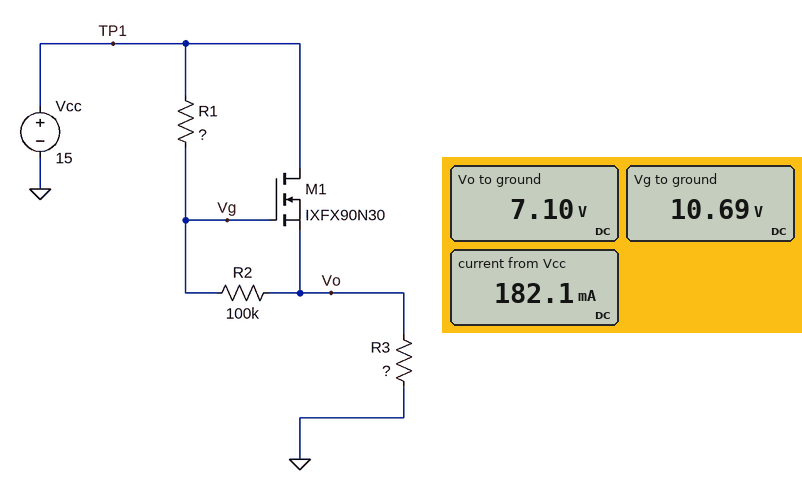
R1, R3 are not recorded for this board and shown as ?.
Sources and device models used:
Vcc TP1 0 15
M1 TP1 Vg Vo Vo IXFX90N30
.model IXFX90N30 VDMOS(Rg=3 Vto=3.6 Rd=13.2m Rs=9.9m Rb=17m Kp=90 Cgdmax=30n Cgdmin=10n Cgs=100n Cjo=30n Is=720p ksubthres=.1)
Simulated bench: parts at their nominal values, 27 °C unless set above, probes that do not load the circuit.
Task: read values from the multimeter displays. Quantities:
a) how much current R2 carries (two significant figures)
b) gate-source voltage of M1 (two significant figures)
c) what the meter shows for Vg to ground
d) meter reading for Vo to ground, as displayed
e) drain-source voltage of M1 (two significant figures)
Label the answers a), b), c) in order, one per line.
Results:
a) 36 µA
b) 3.6 V
c) 10.69 V
d) 7.10 V
e) 7.9 V
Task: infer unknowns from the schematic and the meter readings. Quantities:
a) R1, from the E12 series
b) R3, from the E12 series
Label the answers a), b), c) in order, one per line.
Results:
a) 120 kΩ
b) 39 Ω
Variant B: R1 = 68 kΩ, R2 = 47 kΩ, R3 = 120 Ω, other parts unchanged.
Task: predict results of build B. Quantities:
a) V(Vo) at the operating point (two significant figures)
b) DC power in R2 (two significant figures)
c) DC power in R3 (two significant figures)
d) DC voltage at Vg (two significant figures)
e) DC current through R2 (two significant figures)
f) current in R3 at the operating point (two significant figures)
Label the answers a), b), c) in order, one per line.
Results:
a) 6.4 V
b) 260 µW
c) 340 mW
d) 9.9 V
e) 75 µA
f) 53 mA
